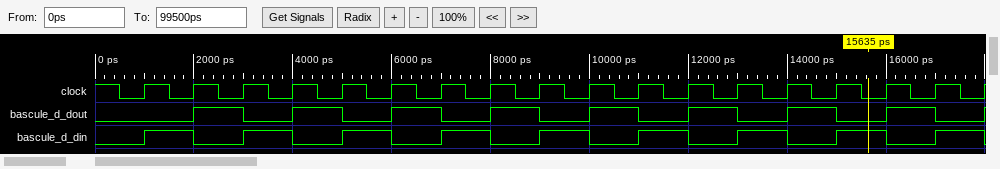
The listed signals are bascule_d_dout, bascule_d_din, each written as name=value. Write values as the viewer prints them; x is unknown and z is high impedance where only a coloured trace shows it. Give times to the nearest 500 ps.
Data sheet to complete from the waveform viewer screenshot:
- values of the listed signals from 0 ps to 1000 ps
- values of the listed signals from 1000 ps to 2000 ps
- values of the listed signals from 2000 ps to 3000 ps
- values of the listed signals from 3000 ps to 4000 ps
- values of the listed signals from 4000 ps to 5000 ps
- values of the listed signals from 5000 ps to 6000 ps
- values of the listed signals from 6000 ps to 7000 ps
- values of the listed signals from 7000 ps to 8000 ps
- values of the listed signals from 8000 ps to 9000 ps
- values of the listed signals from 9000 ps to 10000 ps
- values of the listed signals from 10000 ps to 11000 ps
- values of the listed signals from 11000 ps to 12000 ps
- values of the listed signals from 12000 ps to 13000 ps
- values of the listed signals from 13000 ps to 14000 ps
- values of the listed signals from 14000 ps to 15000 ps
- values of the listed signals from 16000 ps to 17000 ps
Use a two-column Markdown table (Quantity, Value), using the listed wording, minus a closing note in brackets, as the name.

| Quantity | Value |
|---|---|
| values of the listed signals from 0 ps to 1000 ps | bascule_d_dout=0, bascule_d_din=0 |
| values of the listed signals from 1000 ps to 2000 ps | bascule_d_dout=0, bascule_d_din=1 |
| values of the listed signals from 2000 ps to 3000 ps | bascule_d_dout=1, bascule_d_din=0 |
| values of the listed signals from 3000 ps to 4000 ps | bascule_d_dout=0, bascule_d_din=1 |
| values of the listed signals from 4000 ps to 5000 ps | bascule_d_dout=1, bascule_d_din=0 |
| values of the listed signals from 5000 ps to 6000 ps | bascule_d_dout=0, bascule_d_din=1 |
| values of the listed signals from 6000 ps to 7000 ps | bascule_d_dout=1, bascule_d_din=0 |
| values of the listed signals from 7000 ps to 8000 ps | bascule_d_dout=0, bascule_d_din=1 |
| values of the listed signals from 8000 ps to 9000 ps | bascule_d_dout=1, bascule_d_din=0 |
| values of the listed signals from 9000 ps to 10000 ps | bascule_d_dout=0, bascule_d_din=1 |
| values of the listed signals from 10000 ps to 11000 ps | bascule_d_dout=1, bascule_d_din=0 |
| values of the listed signals from 11000 ps to 12000 ps | bascule_d_dout=0, bascule_d_din=1 |
| values of the listed signals from 12000 ps to 13000 ps | bascule_d_dout=1, bascule_d_din=0 |
| values of the listed signals from 13000 ps to 14000 ps | bascule_d_dout=0, bascule_d_din=1 |
| values of the listed signals from 14000 ps to 15000 ps | bascule_d_dout=1, bascule_d_din=0 |
| values of the listed signals from 16000 ps to 17000 ps | bascule_d_dout=1, bascule_d_din=0 |
